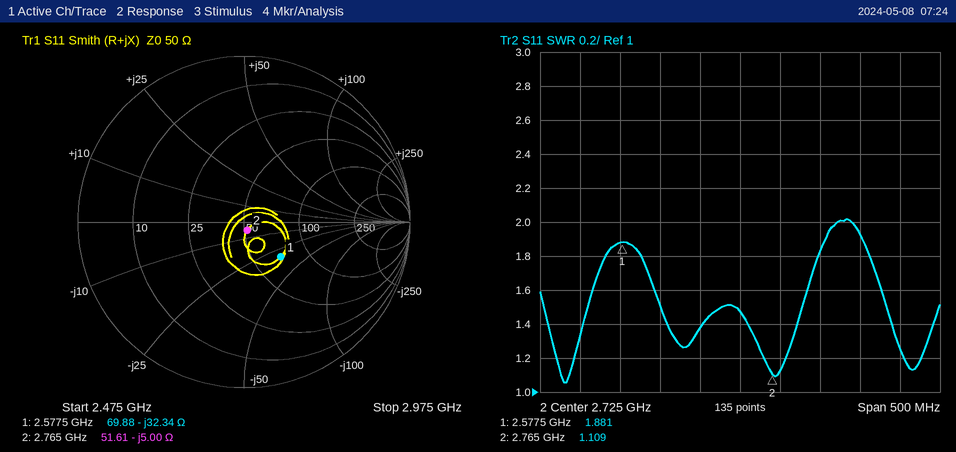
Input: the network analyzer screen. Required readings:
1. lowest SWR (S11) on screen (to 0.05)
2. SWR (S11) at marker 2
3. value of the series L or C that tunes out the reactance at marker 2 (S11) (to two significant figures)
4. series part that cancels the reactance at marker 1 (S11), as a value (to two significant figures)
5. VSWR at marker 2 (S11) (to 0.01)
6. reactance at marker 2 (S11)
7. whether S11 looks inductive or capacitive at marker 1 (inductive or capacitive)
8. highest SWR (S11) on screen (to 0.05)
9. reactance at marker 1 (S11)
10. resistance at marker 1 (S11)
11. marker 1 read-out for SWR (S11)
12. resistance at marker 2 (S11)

1.05
1.109
290 pH
2.0 nH
1.11
-5.00 Ω
capacitive
2.00
-32.34 Ω
69.88 Ω
1.881
51.61 Ω
